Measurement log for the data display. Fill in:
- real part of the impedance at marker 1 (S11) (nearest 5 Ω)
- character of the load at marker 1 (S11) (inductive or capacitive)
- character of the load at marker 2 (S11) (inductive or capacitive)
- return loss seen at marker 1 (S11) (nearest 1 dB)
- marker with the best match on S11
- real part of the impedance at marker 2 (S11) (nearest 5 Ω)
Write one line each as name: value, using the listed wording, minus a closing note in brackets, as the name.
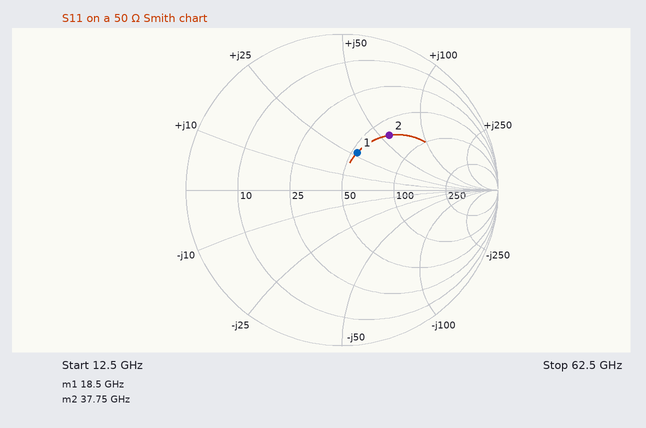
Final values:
real part of the impedance at marker 1 (S11): 55 Ω
character of the load at marker 1 (S11): inductive
character of the load at marker 2 (S11): inductive
return loss seen at marker 1 (S11): 12 dB
marker with the best match on S11: marker 1
real part of the impedance at marker 2 (S11): 65 Ω
